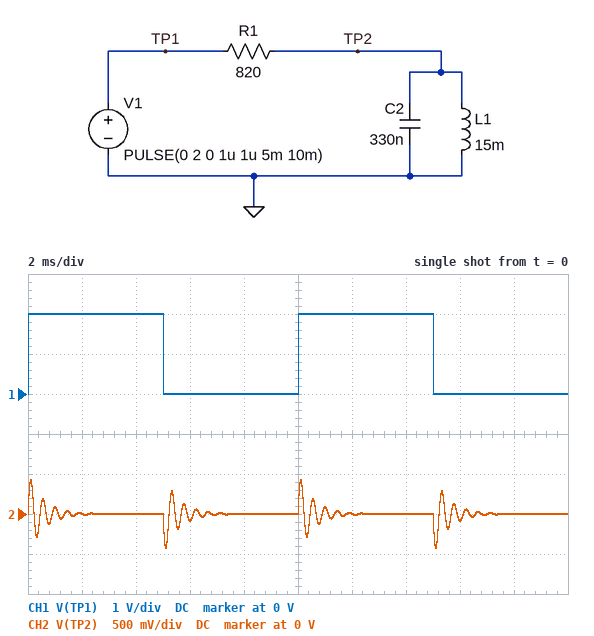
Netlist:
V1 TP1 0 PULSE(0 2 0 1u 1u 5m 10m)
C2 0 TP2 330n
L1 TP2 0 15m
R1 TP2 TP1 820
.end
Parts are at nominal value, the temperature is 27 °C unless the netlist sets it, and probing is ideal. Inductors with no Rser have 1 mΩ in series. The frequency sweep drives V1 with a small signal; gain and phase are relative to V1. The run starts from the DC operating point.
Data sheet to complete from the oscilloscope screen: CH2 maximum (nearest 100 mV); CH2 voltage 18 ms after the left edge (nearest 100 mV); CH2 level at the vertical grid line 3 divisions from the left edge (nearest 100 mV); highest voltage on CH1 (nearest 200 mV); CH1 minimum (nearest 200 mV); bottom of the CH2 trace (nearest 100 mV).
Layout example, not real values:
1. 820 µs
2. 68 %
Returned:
1. 400 mV
2. 0 V
3. -100 mV
4. 2.0 V
5. 0 V
6. -400 mV
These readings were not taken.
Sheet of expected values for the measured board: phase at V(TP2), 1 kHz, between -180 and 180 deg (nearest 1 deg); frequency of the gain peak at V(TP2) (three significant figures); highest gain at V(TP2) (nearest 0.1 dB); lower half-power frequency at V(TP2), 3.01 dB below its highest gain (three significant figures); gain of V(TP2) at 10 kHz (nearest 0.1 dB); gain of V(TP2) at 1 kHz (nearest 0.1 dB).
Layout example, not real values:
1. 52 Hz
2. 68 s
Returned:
1. 82 deg
2. 2.26 kHz
3. 0 dB
4. 1.99 kHz
5. -24.2 dB
6. -17.0 dB
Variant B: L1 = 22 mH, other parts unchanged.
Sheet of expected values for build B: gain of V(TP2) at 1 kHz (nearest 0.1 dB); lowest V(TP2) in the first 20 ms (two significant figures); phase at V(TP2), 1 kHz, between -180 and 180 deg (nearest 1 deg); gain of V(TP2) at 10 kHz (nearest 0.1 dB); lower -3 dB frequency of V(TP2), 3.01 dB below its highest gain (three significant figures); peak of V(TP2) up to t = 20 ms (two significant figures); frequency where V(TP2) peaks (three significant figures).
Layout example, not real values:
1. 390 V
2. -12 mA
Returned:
1. -12.8 dB
2. -500 mV
3. 77 deg
4. -24.3 dB
5. 1.60 kHz
6. 500 mV
7. 1.87 kHz
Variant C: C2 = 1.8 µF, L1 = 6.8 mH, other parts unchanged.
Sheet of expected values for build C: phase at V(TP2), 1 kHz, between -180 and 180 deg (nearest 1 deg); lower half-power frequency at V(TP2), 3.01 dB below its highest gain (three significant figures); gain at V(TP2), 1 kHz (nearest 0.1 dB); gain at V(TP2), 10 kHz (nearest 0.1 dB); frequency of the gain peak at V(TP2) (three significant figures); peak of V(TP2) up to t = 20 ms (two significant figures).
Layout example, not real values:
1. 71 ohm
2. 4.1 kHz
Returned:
1. 84 deg
2. 1.39 kHz
3. -20.0 dB
4. -39.2 dB
5. 1.44 kHz
6. 140 mV
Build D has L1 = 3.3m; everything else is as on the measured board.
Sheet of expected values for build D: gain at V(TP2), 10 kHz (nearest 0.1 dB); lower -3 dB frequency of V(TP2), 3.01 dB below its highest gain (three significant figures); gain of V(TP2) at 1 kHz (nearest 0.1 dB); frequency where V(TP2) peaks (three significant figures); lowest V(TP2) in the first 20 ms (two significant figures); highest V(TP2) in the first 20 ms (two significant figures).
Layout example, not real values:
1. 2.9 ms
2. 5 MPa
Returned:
1. -22.3 dB
2. 4.54 kHz
3. -31.6 dB
4. 4.82 kHz
5. -220 mV
6. 220 mV
